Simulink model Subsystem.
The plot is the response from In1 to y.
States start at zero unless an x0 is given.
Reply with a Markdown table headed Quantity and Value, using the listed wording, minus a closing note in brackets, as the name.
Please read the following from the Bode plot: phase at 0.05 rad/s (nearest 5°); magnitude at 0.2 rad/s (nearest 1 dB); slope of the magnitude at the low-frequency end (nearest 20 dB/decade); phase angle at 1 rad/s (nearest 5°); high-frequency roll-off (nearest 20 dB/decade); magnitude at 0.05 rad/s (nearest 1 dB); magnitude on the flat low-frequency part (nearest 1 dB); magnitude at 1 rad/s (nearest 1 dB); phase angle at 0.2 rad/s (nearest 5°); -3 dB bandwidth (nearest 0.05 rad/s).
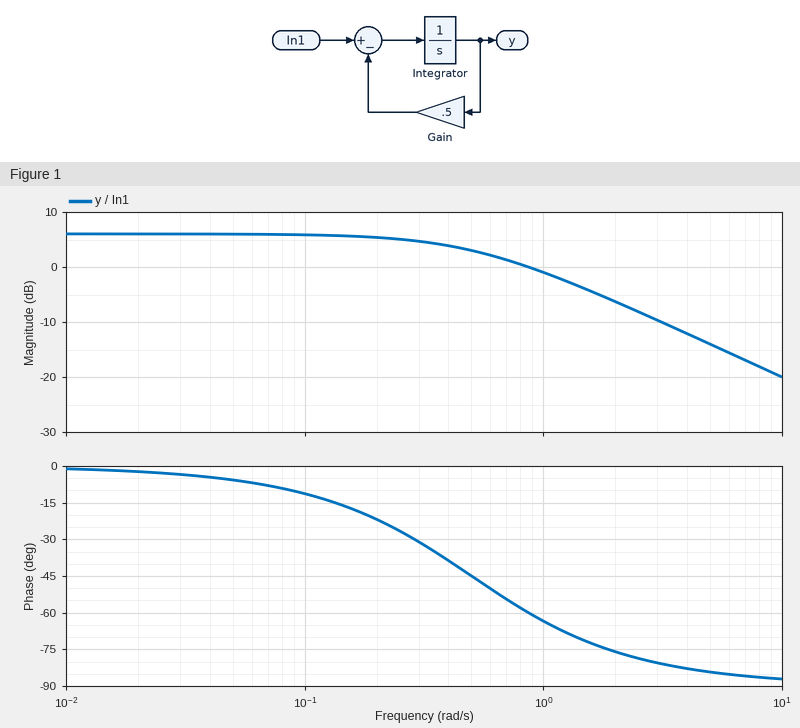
| Quantity | Value |
|---|---|
| phase at 0.05 rad/s | -5° |
| magnitude at 0.2 rad/s | 5 dB |
| slope of the magnitude at the low-frequency end | 0 dB/decade |
| phase angle at 1 rad/s | -65° |
| high-frequency roll-off | -20 dB/decade |
| magnitude at 0.05 rad/s | 6 dB |
| magnitude on the flat low-frequency part | 6 dB |
| magnitude at 1 rad/s | -1 dB |
| phase angle at 0.2 rad/s | -20° |
| -3 dB bandwidth | 0.50 rad/s |
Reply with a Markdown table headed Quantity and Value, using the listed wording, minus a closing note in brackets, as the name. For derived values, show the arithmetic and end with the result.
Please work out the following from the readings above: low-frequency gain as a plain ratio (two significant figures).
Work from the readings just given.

| Quantity | Value |
|---|---|
| low-frequency gain as a plain ratio | 10^(6 / 20) = 2.0 |
